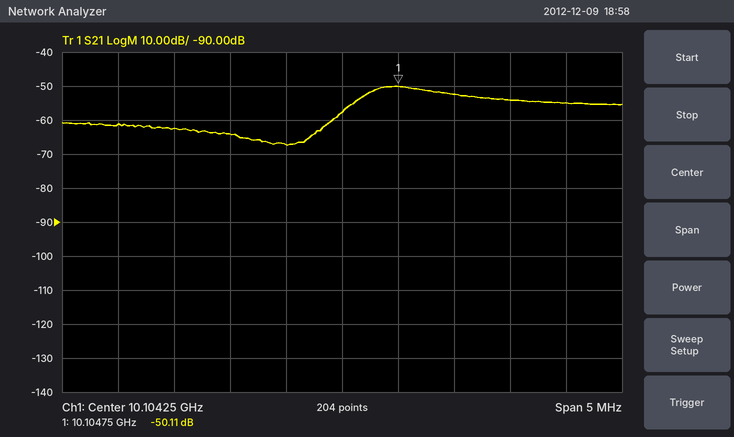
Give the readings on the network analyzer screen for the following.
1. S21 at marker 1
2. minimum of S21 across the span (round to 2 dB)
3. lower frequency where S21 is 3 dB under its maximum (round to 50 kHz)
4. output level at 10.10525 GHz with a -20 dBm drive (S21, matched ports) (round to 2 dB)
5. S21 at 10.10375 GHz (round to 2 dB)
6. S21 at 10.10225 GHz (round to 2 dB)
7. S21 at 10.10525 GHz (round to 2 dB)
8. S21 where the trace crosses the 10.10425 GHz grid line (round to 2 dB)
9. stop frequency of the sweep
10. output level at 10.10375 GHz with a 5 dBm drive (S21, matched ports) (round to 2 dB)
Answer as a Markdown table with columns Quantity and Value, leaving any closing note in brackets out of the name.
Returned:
| Quantity | Value |
|---|---|
| S21 at marker 1 | -50.11 dB |
| minimum of S21 across the span | -68 dB |
| lower frequency where S21 is 3 dB under its maximum | 10.10445 GHz |
| output level at 10.10525 GHz with a -20 dBm drive (S21, matched ports) | -72 dBm |
| S21 at 10.10375 GHz | -68 dB |
| S21 at 10.10225 GHz | -62 dB |
| S21 at 10.10525 GHz | -52 dB |
| S21 where the trace crosses the 10.10425 GHz grid line | -58 dB |
| stop frequency of the sweep | 10.10675 GHz |
| output level at 10.10375 GHz with a 5 dBm drive (S21, matched ports) | -62 dBm |
